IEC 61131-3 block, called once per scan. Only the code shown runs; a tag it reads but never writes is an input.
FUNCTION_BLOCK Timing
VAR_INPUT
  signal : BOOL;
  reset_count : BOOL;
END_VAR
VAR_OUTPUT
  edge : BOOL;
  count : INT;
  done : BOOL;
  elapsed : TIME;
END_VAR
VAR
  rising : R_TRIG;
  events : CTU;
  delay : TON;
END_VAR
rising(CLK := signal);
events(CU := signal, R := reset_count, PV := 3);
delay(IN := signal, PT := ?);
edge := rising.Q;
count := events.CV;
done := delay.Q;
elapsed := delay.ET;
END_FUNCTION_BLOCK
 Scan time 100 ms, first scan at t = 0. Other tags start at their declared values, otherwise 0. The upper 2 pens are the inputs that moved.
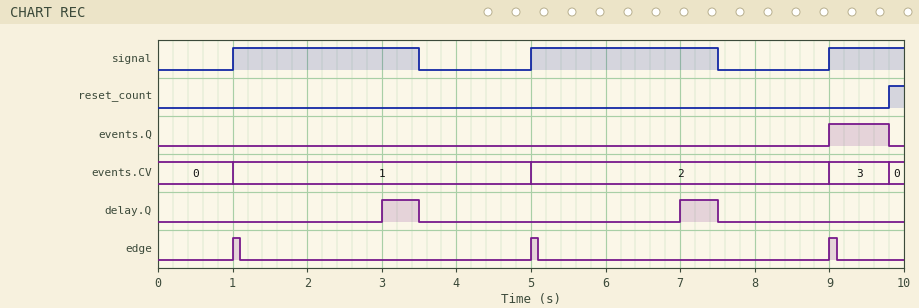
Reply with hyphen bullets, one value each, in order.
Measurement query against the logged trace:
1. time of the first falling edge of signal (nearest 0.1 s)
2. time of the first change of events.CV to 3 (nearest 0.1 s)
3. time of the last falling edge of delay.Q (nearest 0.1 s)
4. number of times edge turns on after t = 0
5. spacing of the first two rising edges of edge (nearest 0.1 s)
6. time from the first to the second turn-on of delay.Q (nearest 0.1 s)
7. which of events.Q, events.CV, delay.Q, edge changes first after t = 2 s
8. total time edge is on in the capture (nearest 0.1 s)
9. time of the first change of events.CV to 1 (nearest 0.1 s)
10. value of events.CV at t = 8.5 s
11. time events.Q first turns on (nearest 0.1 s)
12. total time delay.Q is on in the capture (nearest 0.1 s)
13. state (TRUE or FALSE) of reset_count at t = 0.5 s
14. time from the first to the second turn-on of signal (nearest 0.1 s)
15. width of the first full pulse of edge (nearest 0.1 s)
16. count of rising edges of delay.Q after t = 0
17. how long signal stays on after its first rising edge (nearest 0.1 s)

- 3.5 s
- 9.0 s
- 7.5 s
- 3
- 4.0 s
- 4.0 s
- delay.Q
- 0.3 s
- 1.0 s
- 2
- 9.0 s
- 1.0 s
- FALSE
- 4.0 s
- 0.1 s
- 2
- 2.5 s
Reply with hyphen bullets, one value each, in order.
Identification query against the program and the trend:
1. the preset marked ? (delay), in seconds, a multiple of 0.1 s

- 2.0 s
